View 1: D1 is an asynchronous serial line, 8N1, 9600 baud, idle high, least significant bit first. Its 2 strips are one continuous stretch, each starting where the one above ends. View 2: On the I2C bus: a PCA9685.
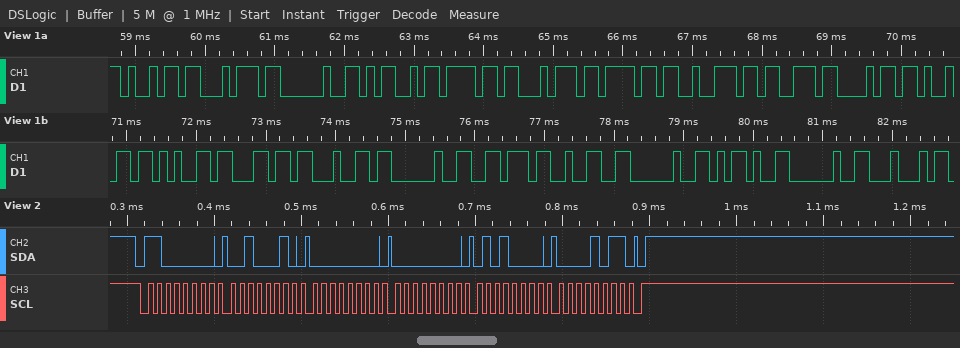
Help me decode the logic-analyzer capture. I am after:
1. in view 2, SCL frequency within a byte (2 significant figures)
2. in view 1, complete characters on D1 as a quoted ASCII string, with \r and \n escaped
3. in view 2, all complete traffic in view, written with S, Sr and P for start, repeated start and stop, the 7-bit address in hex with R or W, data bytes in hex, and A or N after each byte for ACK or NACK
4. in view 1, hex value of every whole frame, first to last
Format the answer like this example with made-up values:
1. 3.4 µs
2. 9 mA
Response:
1. 100 kHz
2. "it Motorshield v2 - D"
3. S 60W A 22 A 00 A 00 A 50 A 0B A P
4. 69 74 20 4D 6F 74 6F 72 73 68 69 65 6C 64 20 76 32 20 2D 20 44
